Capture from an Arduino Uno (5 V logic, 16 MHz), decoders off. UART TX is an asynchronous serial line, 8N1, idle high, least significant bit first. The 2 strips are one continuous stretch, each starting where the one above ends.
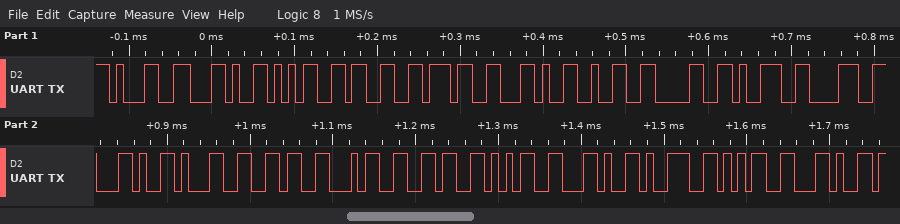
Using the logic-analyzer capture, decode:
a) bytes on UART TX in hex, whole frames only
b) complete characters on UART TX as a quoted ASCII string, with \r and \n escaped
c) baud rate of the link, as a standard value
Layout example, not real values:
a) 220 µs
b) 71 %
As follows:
a) 0x31 0x2C 0x35 0x33 0x37 0x2C 0x32 0x30 0x39 0x38 0x2C 0x31 0x36 0x34 0x36 0x35 0x2C 0x39 0x35 0x2C
b) "1,537,2098,16465,95,"
c) 115200 baud
